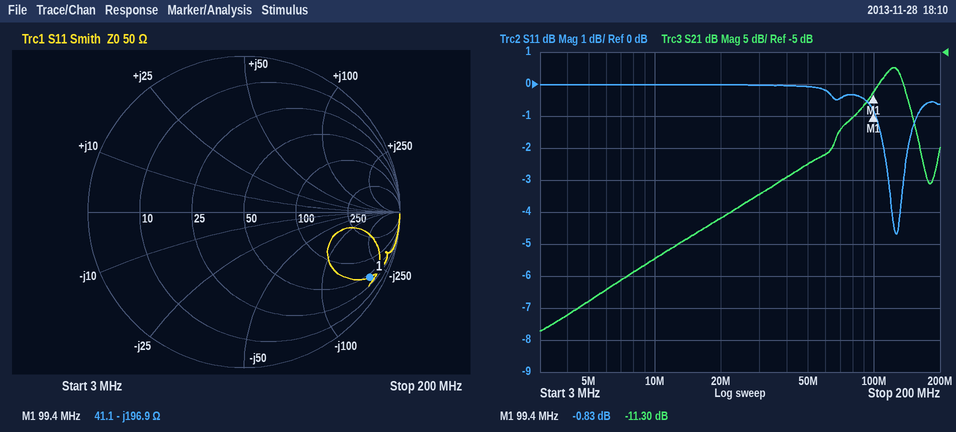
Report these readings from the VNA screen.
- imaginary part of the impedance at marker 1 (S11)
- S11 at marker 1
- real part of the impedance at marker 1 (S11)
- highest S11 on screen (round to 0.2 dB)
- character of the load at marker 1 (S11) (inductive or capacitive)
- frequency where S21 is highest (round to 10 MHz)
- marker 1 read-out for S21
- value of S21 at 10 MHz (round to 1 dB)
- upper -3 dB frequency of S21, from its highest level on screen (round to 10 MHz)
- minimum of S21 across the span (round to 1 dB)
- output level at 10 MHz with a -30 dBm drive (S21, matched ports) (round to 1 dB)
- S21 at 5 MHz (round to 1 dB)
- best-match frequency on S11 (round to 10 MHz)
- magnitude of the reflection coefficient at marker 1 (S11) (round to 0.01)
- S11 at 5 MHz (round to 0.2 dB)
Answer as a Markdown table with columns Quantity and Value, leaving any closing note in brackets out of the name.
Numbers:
| Quantity | Value |
|---|---|
| imaginary part of the impedance at marker 1 | -196.9 Ω |
| S11 at marker 1 | -0.83 dB |
| real part of the impedance at marker 1 | 41.1 Ω |
| highest S11 on screen | 0.0 dB |
| character of the load at marker 1 (S11) | capacitive |
| frequency where S21 is highest | 120 MHz |
| marker 1 read-out for S21 | -11.30 dB |
| value of S21 at 10 MHz | -37 dB |
| upper -3 dB frequency of S21, from its highest level on screen | 140 MHz |
| minimum of S21 across the span | -49 dB |
| output level at 10 MHz with a -30 dBm drive (S21, matched ports) | -67 dBm |
| S21 at 5 MHz | -44 dB |
| best-match frequency on S11 | 130 MHz |
| magnitude of the reflection coefficient at marker 1 (S11) | 0.91 |
| S11 at 5 MHz | 0.0 dB |
